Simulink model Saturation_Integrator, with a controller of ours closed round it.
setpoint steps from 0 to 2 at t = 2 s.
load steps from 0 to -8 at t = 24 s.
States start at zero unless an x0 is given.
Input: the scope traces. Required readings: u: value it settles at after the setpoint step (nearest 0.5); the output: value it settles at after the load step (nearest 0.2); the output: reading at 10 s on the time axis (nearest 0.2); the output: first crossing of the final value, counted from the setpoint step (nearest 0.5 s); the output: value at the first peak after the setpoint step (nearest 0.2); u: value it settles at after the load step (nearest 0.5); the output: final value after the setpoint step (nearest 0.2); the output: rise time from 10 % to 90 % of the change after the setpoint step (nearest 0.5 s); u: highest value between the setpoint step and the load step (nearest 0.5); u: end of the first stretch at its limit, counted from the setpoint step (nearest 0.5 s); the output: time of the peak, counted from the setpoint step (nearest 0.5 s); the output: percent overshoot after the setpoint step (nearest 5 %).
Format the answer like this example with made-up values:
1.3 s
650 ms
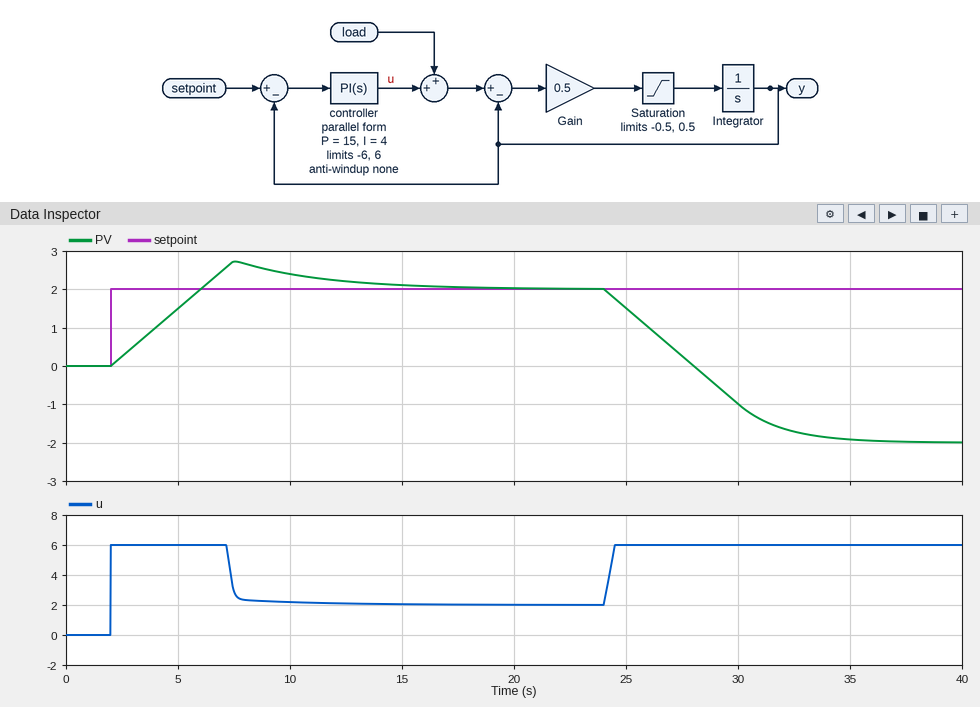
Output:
2.0
-2.0
2.4
4.0 s
2.8
6.0
2.0
3.0 s
6.0
5.0 s
5.5 s
35 %
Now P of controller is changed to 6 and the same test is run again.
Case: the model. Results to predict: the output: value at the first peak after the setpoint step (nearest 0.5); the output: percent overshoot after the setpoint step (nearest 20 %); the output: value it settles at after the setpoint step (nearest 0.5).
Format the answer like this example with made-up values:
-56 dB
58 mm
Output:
3.0
60 %
2.0
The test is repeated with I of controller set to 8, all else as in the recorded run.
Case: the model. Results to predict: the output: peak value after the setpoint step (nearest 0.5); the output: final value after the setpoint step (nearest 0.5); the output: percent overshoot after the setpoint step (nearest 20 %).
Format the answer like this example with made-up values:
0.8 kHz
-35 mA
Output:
3.0
2.0
60 %
